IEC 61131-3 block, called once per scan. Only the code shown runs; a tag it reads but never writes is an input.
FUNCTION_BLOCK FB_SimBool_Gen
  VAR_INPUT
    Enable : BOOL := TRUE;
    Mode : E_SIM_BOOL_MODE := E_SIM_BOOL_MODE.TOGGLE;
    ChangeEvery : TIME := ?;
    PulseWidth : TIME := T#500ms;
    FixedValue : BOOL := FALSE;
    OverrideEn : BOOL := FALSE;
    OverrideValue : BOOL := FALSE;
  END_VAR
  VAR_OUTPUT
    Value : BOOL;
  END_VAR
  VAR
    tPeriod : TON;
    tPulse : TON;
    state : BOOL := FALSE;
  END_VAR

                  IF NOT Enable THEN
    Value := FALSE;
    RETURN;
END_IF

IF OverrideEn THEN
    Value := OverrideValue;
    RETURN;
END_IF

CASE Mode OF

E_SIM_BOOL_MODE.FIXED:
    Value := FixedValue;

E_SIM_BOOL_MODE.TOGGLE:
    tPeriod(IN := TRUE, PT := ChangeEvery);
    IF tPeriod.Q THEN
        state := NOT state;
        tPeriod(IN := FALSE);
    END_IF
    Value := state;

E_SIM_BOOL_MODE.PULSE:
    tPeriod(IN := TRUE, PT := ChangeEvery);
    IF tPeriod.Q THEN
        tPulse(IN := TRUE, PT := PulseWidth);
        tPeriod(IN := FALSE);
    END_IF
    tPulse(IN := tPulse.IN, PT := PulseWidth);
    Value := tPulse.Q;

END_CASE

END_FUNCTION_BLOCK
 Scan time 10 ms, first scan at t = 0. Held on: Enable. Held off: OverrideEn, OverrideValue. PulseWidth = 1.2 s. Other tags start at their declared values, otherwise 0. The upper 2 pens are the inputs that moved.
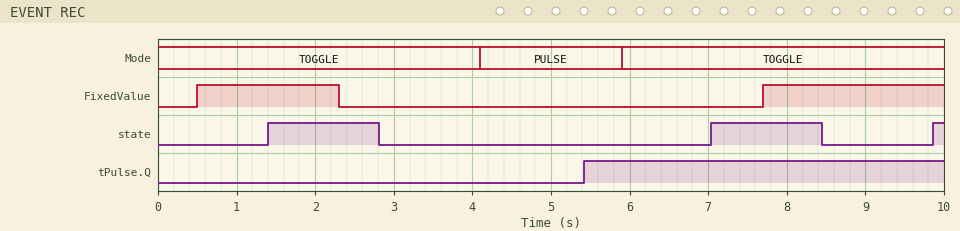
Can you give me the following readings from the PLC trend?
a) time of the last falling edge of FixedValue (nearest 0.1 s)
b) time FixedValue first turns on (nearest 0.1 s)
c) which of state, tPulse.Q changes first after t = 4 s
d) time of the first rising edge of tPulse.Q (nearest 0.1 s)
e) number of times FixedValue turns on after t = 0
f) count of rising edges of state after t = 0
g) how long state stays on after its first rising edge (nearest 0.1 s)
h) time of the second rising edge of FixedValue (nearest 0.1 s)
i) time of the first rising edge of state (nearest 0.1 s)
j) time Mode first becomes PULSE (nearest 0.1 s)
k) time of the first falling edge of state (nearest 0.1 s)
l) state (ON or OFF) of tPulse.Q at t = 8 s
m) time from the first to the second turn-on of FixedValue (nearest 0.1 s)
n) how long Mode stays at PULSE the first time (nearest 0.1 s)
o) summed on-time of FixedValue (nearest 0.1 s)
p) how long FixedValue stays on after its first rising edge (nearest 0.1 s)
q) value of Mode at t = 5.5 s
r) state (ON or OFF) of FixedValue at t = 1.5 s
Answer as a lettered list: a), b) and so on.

a) 2.3 s
b) 0.5 s
c) tPulse.Q
d) 5.4 s
e) 2
f) 3
g) 1.4 s
h) 7.7 s
i) 1.4 s
j) 4.1 s
k) 2.8 s
l) ON
m) 7.2 s
n) 1.8 s
o) 4.1 s
p) 1.8 s
q) PULSE
r) ON
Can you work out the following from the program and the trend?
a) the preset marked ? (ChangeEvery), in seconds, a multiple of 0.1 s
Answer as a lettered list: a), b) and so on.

a) 1.4 s
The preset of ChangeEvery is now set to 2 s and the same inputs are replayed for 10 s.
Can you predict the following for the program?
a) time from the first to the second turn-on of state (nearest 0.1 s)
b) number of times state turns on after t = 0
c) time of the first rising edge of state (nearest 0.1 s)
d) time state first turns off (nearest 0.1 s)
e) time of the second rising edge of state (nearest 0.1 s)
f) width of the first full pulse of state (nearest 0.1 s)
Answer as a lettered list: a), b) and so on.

a) 4.0 s
b) 2
c) 2.0 s
d) 4.0 s
e) 6.0 s
f) 2.0 s
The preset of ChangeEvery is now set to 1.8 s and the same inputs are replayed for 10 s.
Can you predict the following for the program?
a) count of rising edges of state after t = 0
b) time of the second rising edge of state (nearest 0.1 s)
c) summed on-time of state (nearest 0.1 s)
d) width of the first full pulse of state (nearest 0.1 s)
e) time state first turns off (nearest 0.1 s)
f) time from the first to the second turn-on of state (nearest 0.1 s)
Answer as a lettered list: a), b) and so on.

a) 2
b) 7.2 s
c) 3.6 s
d) 1.8 s
e) 3.6 s
f) 5.4 s
